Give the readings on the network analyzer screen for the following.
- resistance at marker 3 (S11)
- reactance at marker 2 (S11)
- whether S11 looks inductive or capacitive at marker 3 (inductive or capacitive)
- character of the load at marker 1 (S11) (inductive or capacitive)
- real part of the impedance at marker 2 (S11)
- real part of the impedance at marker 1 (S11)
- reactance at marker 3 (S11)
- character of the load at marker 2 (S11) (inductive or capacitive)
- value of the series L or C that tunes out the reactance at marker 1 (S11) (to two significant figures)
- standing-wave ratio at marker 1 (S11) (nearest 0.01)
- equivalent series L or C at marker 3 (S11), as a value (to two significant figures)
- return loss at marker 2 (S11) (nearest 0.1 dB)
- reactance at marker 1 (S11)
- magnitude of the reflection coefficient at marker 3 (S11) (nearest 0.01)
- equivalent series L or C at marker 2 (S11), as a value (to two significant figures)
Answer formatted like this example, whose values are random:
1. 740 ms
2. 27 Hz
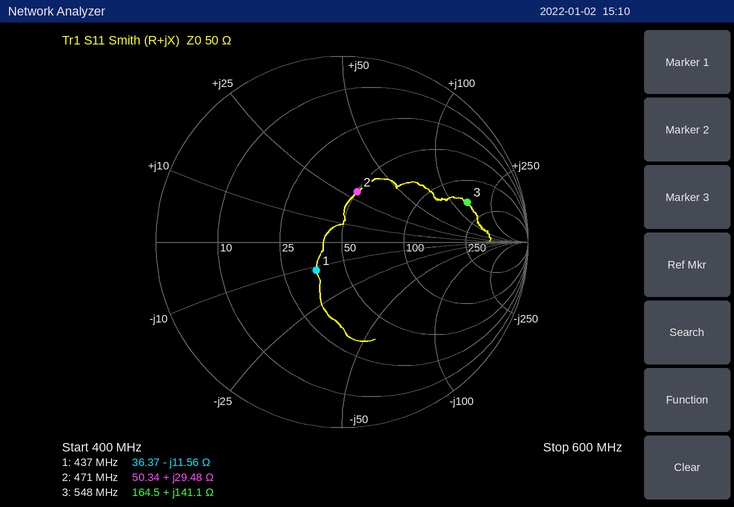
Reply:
1. 164.5 Ω
2. +29.48 Ω
3. inductive
4. capacitive
5. 50.34 Ω
6. 36.37 Ω
7. +141.1 Ω
8. inductive
9. 4.2 nH
10. 1.52
11. 41 nH
12. 11.0 dB
13. -11.56 Ω
14. 0.71
15. 10.0 nH
